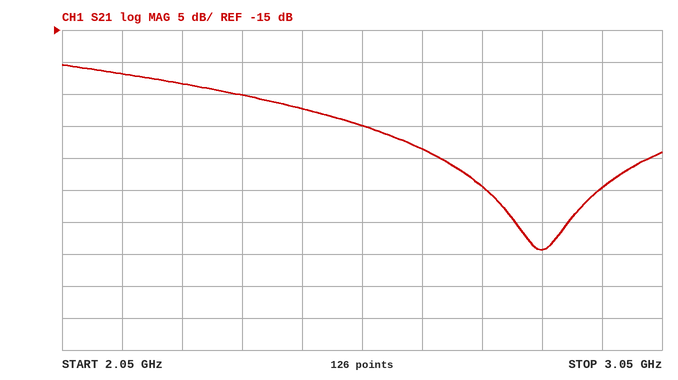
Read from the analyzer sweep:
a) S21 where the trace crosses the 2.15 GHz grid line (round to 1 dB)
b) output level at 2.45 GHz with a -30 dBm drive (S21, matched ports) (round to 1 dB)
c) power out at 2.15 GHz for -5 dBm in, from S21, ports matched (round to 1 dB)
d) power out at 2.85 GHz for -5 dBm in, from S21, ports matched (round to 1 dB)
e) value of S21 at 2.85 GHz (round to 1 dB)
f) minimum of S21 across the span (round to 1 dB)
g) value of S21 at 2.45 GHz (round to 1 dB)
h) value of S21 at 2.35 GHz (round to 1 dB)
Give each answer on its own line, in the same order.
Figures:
-22 dB
-57 dBm
-27 dBm
-54 dBm
-49 dB
-49 dB
-27 dB
-25 dB
